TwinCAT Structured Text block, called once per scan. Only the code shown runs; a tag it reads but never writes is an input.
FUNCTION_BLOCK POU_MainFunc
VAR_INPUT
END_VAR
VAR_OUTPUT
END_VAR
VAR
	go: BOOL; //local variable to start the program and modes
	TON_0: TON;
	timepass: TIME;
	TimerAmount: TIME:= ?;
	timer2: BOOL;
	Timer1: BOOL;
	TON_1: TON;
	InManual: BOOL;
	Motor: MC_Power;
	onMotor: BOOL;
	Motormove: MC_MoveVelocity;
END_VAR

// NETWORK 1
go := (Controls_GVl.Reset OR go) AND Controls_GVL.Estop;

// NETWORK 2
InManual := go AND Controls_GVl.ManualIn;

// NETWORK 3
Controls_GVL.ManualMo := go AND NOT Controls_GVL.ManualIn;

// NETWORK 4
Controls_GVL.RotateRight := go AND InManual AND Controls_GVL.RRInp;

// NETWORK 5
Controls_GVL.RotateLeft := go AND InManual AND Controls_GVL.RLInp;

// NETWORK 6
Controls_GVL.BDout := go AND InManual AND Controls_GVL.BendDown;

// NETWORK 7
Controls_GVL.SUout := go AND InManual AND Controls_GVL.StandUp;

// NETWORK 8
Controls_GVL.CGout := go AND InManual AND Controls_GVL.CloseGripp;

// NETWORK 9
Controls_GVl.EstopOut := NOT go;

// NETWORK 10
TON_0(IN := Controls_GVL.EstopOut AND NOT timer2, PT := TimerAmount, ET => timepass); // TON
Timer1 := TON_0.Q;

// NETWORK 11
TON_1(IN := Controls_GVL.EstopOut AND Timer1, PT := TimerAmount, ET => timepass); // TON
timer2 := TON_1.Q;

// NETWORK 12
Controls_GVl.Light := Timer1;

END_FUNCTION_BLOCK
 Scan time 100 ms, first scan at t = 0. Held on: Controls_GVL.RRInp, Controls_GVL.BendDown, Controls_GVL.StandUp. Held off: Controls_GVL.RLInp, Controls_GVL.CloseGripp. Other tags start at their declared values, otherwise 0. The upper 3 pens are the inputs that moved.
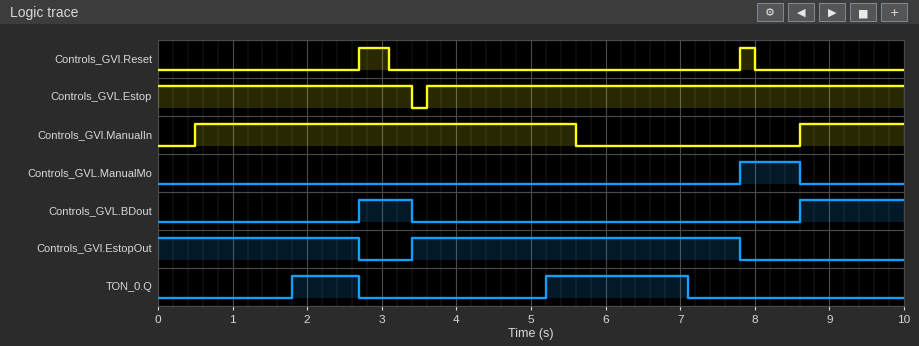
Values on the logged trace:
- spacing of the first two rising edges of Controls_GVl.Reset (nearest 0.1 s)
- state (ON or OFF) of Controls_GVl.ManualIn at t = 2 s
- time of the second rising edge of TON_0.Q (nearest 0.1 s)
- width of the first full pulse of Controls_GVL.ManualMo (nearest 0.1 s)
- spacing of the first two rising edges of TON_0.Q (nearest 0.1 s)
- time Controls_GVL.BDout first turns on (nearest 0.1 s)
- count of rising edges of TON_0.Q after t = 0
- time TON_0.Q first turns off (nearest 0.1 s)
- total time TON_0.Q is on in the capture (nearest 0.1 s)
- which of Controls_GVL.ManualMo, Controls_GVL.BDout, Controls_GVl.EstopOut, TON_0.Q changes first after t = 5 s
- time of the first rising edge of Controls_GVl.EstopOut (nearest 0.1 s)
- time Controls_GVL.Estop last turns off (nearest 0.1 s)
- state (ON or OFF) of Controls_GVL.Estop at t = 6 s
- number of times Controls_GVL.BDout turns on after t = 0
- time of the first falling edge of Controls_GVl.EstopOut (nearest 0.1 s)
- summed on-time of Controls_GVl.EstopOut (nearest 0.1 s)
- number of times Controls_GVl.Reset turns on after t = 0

5.1 s
ON
5.2 s
0.8 s
3.4 s
2.7 s
2
2.7 s
2.8 s
TON_0.Q
3.4 s
3.4 s
ON
2
2.7 s
7.1 s
2
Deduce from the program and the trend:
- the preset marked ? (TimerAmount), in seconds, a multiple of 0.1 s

1.8 s
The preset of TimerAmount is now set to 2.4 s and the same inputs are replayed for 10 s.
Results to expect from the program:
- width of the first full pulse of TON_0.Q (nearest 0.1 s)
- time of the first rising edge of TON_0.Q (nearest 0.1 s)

0.3 s
2.4 s
